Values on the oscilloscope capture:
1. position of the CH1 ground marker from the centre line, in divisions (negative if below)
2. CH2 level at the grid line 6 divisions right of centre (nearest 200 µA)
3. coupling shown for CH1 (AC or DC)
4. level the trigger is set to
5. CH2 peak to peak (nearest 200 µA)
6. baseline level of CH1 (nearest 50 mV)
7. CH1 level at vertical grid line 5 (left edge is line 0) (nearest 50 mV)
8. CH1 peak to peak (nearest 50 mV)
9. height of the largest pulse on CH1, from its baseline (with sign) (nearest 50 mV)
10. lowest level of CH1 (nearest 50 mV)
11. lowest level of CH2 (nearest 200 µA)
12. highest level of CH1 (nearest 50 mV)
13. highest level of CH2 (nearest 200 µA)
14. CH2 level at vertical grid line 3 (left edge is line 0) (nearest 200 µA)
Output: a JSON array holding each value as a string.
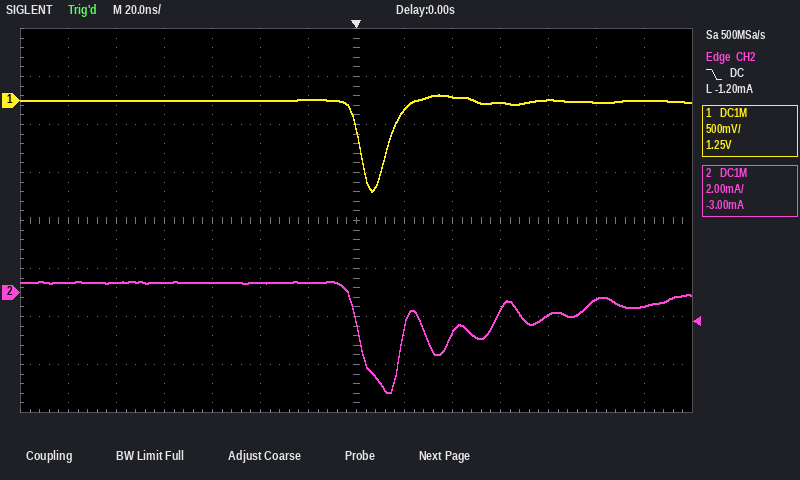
["+2.5 div", "-600 µA", "DC", "-1.20 mA", "4.6 mA", "0 mV", "0 mV", "1.00 V", "-950 mV", "-950 mV", "-4.2 mA", "50 mV", "400 µA", "400 µA"]
